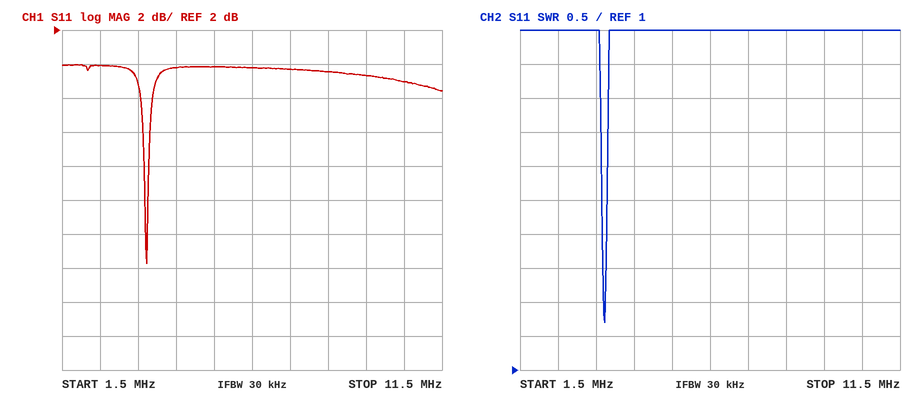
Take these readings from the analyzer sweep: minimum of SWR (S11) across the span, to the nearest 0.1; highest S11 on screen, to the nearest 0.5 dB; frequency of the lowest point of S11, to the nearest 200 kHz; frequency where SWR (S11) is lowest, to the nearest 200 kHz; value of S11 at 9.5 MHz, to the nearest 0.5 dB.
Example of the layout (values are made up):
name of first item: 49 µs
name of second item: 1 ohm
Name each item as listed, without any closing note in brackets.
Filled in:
minimum of SWR (S11) across the span, to the nearest 0.1: 1.7
highest S11 on screen, to the nearest 0.5 dB: 0.0 dB
frequency of the lowest point of S11, to the nearest 200 kHz: 3.8 MHz
frequency where SWR (S11) is lowest, to the nearest 200 kHz: 3.8 MHz
value of S11 at 9.5 MHz, to the nearest 0.5 dB: -0.5 dB
